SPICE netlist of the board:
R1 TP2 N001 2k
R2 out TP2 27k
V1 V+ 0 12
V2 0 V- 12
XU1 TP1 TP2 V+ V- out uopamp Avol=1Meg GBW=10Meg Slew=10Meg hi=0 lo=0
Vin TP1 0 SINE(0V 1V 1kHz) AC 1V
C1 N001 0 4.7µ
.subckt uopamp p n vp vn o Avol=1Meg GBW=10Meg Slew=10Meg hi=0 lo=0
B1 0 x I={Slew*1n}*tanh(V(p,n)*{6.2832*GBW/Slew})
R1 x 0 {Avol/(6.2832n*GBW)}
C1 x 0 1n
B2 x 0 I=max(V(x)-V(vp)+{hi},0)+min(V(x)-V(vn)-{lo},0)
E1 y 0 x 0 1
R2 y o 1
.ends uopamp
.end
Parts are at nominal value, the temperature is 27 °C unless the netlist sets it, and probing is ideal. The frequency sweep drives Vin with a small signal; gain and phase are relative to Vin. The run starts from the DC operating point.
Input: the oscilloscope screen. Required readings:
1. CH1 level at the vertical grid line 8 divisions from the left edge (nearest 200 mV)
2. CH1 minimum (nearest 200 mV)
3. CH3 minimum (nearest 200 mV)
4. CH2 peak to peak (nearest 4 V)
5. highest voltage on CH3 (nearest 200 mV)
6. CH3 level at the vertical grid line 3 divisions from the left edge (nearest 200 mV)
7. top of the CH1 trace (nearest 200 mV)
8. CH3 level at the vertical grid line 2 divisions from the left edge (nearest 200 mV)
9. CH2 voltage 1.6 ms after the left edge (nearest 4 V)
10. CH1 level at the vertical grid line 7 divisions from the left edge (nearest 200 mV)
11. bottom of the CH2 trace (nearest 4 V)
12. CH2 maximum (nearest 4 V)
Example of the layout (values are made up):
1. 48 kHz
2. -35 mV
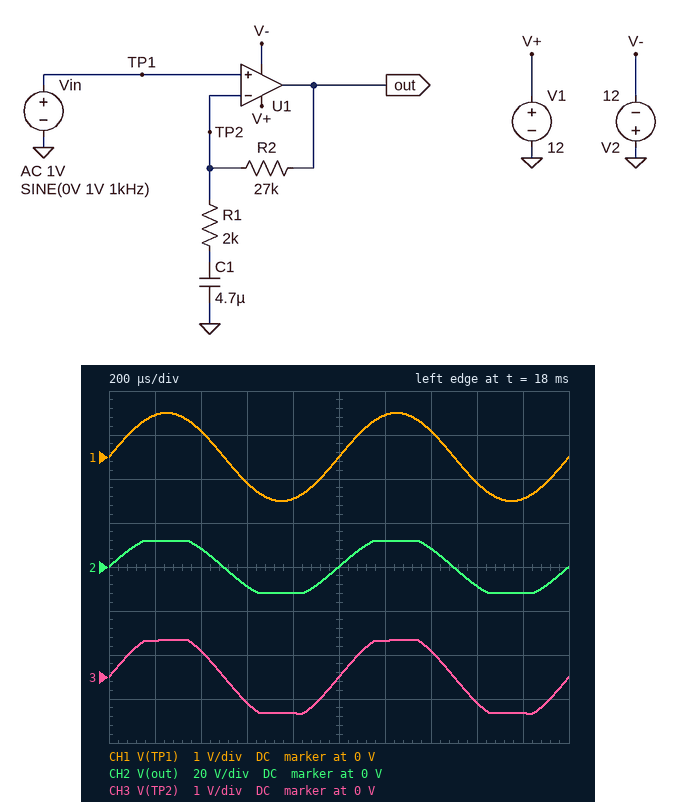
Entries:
1. -600 mV
2. -1.0 V
3. -800 mV
4. 24 V
5. 800 mV
6. -600 mV
7. 1.0 V
8. 600 mV
9. -8 V
10. 600 mV
11. -12 V
12. 12 V
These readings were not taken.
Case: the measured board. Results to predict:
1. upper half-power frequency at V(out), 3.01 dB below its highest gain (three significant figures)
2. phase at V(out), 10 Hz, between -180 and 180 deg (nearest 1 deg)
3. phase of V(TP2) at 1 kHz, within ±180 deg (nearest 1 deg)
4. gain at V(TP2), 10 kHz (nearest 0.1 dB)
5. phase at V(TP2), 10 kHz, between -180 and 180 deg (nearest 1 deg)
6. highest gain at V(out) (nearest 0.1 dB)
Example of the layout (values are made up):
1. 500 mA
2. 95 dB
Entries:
1. 690 kHz
2. 53 deg
3. 0 deg
4. 0 dB
5. -1 deg
6. 23.2 dB
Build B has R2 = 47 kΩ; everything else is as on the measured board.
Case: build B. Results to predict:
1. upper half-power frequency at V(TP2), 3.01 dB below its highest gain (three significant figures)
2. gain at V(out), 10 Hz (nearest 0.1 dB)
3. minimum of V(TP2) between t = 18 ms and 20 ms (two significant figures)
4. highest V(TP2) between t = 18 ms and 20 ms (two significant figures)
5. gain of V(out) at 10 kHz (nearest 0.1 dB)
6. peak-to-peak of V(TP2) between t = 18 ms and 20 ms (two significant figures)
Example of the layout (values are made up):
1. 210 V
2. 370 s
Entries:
1. 408 kHz
2. 21.9 dB
3. -490 mV
4. 500 mV
5. 27.8 dB
6. 1.0 V
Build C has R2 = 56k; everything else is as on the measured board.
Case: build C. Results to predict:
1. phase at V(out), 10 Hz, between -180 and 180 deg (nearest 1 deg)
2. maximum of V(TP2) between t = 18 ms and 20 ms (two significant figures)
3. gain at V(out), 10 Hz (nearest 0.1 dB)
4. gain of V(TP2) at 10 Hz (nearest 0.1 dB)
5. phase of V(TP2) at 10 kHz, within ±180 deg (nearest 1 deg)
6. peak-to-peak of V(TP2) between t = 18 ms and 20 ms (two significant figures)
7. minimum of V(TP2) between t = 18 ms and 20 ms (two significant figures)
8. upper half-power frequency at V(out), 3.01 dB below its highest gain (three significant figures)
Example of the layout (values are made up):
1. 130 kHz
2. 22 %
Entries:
1. 56 deg
2. 430 mV
3. 23.4 dB
4. 0 dB
5. -2 deg
6. 840 mV
7. -420 mV
8. 345 kHz
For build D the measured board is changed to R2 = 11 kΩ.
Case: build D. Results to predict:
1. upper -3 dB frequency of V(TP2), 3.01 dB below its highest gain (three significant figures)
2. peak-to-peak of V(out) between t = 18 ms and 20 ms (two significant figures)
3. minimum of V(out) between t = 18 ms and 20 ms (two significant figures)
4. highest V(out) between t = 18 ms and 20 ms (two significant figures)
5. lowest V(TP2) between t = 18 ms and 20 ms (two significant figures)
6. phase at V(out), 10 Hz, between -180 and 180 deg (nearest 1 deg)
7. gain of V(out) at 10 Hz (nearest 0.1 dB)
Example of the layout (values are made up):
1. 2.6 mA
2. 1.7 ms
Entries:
1. 1.54 MHz
2. 13 V
3. -6.5 V
4. 6.5 V
5. -1.0 V
6. 45 deg
7. 10.7 dB
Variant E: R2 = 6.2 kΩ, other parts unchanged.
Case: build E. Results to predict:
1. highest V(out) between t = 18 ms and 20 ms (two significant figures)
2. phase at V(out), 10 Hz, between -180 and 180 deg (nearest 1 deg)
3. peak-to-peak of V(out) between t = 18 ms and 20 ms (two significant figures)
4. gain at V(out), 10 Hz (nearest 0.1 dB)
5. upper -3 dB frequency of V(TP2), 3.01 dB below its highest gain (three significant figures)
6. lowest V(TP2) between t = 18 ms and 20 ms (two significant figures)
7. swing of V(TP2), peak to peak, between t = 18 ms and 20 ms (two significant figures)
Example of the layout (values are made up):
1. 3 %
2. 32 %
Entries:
1. 4.1 V
2. 37 deg
3. 8.2 V
4. 7.1 dB
5. 2.44 MHz
6. -1.0 V
7. 2.0 V
